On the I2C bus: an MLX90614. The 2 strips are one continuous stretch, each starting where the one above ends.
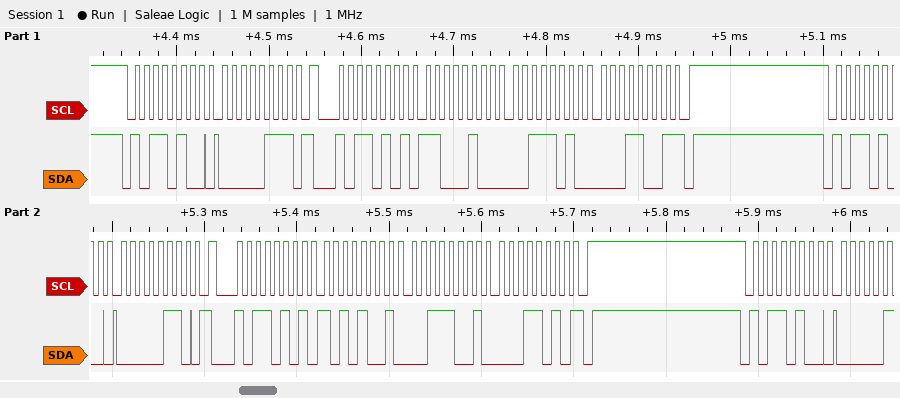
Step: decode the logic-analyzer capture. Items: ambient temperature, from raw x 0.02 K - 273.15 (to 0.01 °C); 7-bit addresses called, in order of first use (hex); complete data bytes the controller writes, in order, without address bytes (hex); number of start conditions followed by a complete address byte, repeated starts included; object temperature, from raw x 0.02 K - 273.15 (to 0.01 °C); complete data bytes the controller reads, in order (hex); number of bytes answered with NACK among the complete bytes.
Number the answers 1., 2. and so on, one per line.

1. 22.07 °C
2. 0x5A
3. 07 06
4. 5
5. 27.73 °C
6. C4 3A 19 A9 39 1A
7. 2
